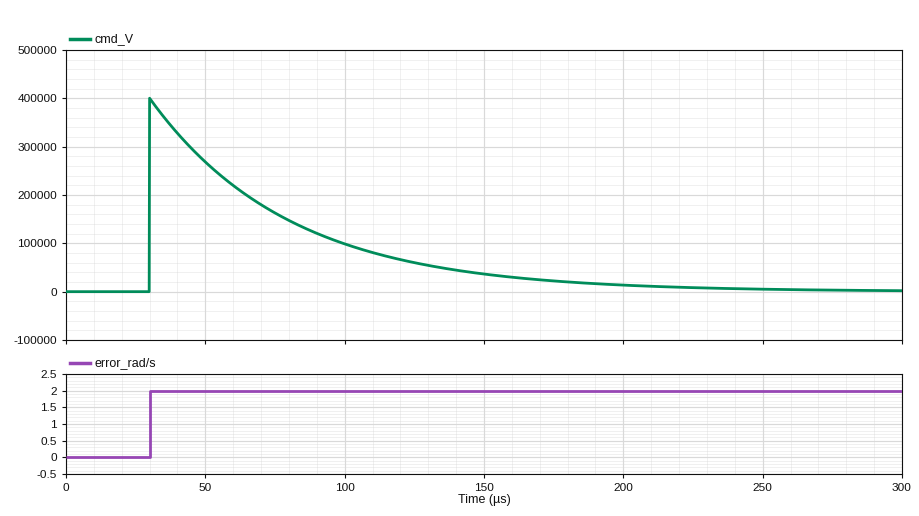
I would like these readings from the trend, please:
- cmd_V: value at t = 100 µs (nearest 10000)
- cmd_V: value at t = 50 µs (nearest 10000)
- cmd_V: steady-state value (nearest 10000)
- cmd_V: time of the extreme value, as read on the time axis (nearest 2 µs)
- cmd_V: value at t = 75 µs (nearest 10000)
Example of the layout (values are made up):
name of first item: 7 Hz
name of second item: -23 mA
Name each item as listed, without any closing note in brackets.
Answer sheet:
cmd_V: value at t = 100 µs: 100000
cmd_V: value at t = 50 µs: 270000
cmd_V: steady-state value: 0
cmd_V: time of the extreme value, as read on the time axis: 30 µs
cmd_V: value at t = 75 µs: 160000
